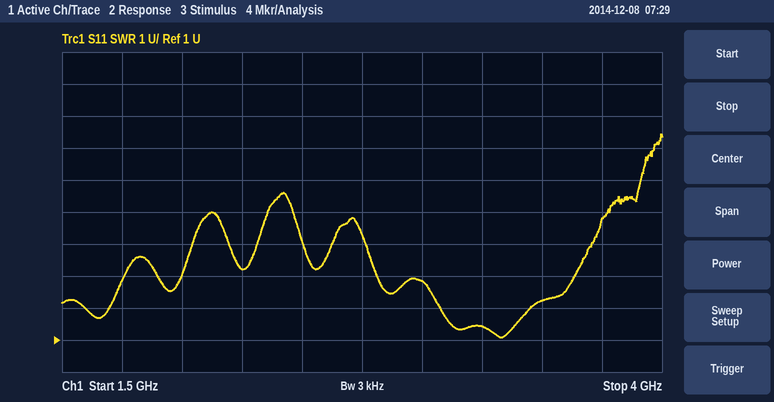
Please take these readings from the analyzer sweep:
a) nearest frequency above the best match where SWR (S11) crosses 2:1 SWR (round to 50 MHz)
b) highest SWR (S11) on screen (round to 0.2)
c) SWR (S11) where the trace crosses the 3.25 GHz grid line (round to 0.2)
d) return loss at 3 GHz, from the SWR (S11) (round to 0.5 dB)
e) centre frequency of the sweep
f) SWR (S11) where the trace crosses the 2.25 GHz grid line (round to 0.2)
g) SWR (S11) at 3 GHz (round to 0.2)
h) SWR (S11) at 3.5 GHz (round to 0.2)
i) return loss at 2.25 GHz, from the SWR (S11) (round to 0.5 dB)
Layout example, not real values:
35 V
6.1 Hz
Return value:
3.45 GHz
7.4
1.4
6.5 dB
2.75 GHz
3.2
2.8
2.2
5.5 dB
